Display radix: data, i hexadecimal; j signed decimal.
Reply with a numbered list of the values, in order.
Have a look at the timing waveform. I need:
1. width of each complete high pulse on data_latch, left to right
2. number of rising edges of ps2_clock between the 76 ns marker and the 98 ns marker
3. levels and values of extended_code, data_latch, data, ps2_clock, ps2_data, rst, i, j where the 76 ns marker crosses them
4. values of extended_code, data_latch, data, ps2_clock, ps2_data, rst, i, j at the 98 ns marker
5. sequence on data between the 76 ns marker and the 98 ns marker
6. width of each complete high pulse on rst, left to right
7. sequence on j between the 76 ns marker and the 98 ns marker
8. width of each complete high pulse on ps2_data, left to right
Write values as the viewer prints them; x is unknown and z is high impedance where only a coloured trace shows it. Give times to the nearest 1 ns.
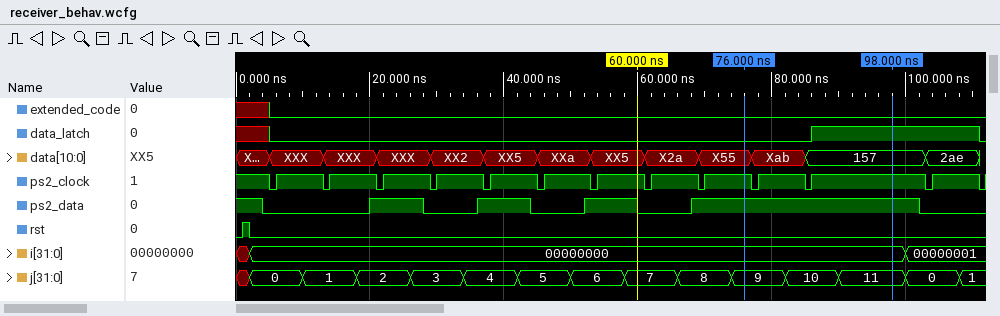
1. 25 ns
2. 2
3. extended_code=0, data_latch=0, data=X55, ps2_clock=1, ps2_data=1, rst=0, i=00000000, j=9
4. extended_code=0, data_latch=1, data=157, ps2_clock=1, ps2_data=1, rst=0, i=00000000, j=11
5. X55, Xab, 157
6. 1 ns
7. 9, 10, 11
8. 8 ns, 8 ns, 8 ns, 34 ns
